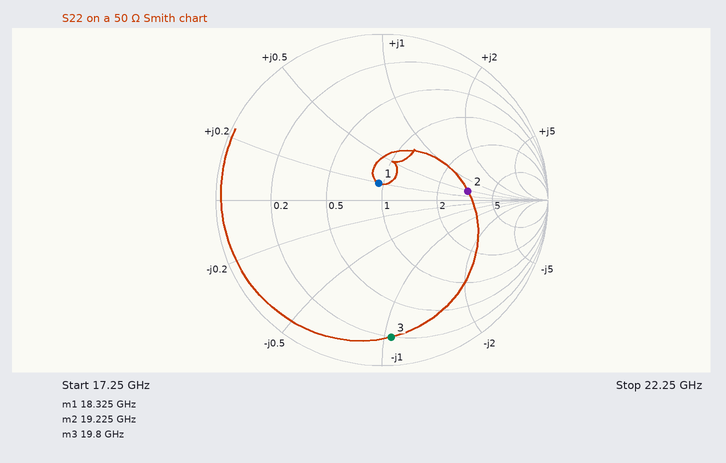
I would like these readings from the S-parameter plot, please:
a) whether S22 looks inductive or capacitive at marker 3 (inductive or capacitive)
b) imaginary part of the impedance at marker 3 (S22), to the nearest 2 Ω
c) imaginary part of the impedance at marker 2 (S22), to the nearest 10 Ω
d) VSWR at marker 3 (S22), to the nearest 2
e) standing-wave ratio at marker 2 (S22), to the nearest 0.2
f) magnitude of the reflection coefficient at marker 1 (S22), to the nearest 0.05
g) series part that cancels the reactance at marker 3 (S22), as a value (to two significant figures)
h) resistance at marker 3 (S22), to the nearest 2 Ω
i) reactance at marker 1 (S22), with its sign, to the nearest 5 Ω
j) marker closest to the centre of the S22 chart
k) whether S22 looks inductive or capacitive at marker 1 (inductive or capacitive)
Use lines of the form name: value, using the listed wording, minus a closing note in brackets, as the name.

whether S22 looks inductive or capacitive at marker 3: capacitive
imaginary part of the impedance at marker 3 (S22), to the nearest 2 Ω: -52 Ω
imaginary part of the impedance at marker 2 (S22), to the nearest 10 Ω: +20 Ω
VSWR at marker 3 (S22), to the nearest 2: 10
standing-wave ratio at marker 2 (S22), to the nearest 0.2: 3.2
magnitude of the reflection coefficient at marker 1 (S22), to the nearest 0.05: 0.10
series part that cancels the reactance at marker 3 (S22), as a value: 420 pH
resistance at marker 3 (S22), to the nearest 2 Ω: 10 Ω
reactance at marker 1 (S22), with its sign, to the nearest 5 Ω: +10 Ω
marker closest to the centre of the S22 chart: marker 1
whether S22 looks inductive or capacitive at marker 1: inductive
